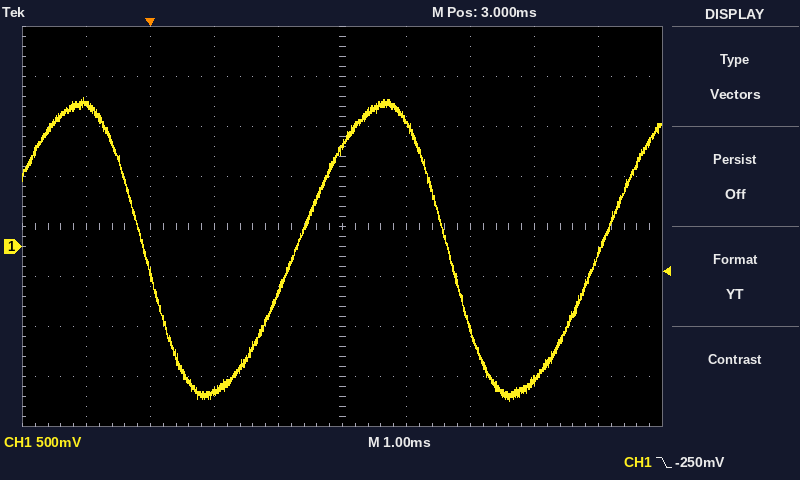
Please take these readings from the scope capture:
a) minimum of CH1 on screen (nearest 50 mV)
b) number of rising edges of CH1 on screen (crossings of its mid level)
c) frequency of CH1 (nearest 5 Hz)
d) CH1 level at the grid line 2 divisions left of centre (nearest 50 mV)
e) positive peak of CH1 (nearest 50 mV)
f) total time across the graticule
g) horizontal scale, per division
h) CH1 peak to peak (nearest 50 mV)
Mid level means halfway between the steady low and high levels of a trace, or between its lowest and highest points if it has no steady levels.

-1.55 V
2
210 Hz
-1.45 V
1.50 V
10 ms
1 ms
3.05 V
